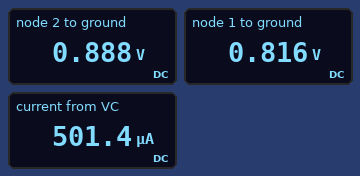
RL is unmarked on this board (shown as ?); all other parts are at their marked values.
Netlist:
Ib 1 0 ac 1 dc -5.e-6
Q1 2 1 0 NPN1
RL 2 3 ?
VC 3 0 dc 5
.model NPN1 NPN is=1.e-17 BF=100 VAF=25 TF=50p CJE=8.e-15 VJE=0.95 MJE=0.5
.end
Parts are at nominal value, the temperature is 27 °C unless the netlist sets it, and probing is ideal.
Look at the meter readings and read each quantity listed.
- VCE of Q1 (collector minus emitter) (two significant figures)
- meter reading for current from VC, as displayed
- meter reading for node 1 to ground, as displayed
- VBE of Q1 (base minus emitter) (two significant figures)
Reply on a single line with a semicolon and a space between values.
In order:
890 mV; 501.4 µA; 0.816 V; 820 mV
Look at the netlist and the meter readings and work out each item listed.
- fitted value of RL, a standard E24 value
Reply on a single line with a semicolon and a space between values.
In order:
8.2 kΩ
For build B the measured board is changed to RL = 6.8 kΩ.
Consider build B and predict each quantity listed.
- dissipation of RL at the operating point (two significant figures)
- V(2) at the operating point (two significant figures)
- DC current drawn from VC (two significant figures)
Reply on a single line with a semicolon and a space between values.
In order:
1.8 mW; 1.5 V; 510 µA
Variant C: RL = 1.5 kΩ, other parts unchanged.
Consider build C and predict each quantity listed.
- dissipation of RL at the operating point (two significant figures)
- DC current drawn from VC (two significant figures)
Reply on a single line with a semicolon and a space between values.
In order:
480 µW; 570 µA
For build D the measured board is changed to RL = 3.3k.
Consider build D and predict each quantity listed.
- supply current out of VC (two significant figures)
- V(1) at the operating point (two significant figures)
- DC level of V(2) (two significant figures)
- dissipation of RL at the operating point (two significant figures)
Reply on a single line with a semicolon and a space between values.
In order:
550 µA; 820 mV; 3.2 V; 990 µW
